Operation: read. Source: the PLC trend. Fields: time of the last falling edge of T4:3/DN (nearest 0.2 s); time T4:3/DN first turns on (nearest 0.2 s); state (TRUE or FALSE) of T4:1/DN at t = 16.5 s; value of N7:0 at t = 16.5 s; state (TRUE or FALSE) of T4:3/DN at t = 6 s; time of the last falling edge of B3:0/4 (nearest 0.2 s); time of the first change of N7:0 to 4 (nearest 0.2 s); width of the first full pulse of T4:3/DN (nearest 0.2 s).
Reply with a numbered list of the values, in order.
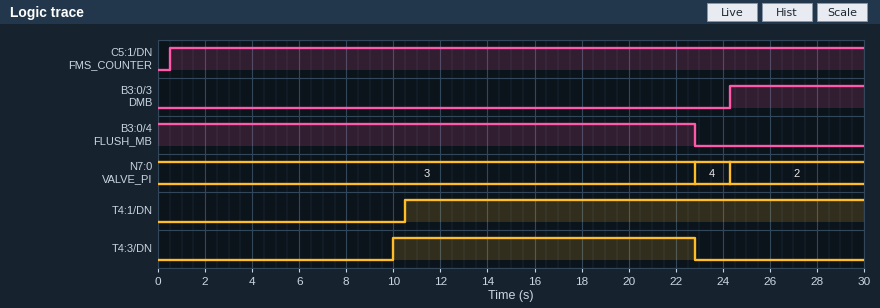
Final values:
1. 22.8 s
2. 10.0 s
3. TRUE
4. 3
5. FALSE
6. 22.8 s
7. 22.8 s
8. 12.8 s
